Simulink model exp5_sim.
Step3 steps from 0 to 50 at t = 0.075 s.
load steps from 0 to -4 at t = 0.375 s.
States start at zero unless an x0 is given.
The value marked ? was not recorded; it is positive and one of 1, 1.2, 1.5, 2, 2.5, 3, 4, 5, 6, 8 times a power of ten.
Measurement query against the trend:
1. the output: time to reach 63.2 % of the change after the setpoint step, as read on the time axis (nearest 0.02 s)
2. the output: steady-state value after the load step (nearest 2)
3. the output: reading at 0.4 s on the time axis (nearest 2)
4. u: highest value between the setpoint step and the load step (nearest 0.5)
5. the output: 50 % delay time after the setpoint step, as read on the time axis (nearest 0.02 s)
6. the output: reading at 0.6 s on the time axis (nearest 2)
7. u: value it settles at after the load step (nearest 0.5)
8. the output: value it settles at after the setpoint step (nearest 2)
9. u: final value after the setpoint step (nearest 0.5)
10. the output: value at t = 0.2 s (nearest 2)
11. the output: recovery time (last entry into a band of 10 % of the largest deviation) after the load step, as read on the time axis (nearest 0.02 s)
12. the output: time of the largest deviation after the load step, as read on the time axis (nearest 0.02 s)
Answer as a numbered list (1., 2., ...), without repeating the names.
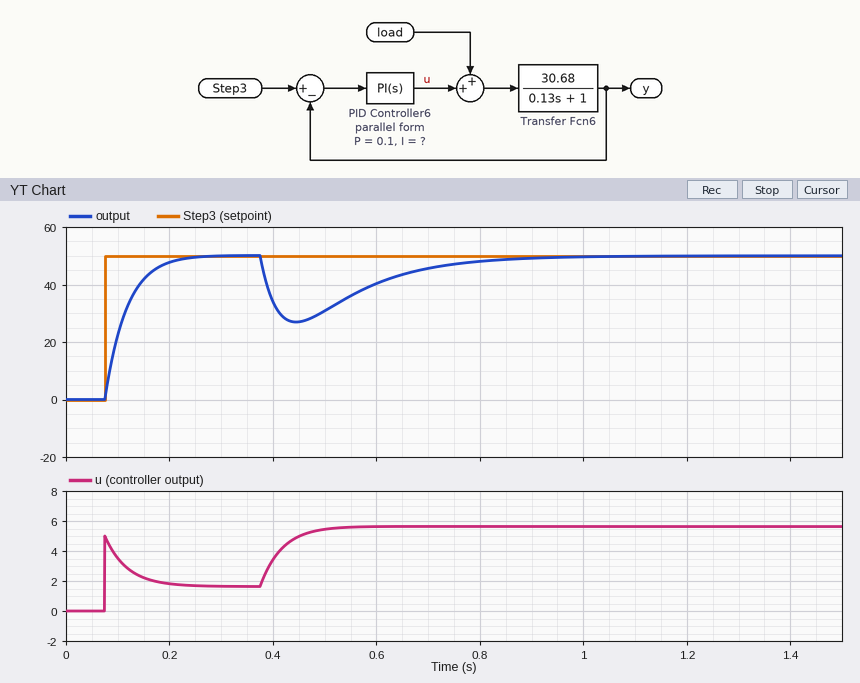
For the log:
1. 0.12 s
2. 50
3. 34
4. 5.0
5. 0.10 s
6. 40
7. 5.5
8. 50
9. 1.5
10. 48
11. 0.78 s
12. 0.44 s
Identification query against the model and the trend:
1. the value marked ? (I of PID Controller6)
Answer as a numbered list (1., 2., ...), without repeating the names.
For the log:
1. 0.8
